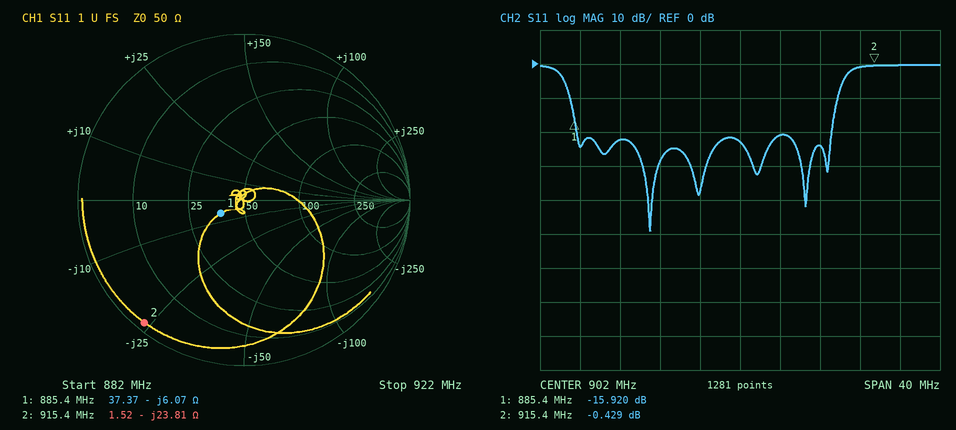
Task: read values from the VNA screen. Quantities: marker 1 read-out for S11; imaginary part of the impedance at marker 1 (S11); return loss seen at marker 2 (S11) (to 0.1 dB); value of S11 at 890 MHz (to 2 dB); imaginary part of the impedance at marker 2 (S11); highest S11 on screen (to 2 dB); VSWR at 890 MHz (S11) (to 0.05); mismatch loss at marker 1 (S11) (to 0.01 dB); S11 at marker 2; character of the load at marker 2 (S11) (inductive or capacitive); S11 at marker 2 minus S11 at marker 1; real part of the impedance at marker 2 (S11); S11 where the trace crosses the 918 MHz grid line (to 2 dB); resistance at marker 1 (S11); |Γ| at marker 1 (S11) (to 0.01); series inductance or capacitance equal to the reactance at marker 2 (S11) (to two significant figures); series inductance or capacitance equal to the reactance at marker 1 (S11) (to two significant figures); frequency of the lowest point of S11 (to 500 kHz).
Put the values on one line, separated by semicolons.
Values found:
-15.920 dB; -6.07 Ω; 0.4 dB; -22 dB; -23.81 Ω; 0 dB; 1.15; 0.11 dB; -0.429 dB; capacitive; 15.491 dB; 1.52 Ω; 0 dB; 37.37 Ω; 0.16; 7.3 pF; 30 pF; 893.0 MHz
